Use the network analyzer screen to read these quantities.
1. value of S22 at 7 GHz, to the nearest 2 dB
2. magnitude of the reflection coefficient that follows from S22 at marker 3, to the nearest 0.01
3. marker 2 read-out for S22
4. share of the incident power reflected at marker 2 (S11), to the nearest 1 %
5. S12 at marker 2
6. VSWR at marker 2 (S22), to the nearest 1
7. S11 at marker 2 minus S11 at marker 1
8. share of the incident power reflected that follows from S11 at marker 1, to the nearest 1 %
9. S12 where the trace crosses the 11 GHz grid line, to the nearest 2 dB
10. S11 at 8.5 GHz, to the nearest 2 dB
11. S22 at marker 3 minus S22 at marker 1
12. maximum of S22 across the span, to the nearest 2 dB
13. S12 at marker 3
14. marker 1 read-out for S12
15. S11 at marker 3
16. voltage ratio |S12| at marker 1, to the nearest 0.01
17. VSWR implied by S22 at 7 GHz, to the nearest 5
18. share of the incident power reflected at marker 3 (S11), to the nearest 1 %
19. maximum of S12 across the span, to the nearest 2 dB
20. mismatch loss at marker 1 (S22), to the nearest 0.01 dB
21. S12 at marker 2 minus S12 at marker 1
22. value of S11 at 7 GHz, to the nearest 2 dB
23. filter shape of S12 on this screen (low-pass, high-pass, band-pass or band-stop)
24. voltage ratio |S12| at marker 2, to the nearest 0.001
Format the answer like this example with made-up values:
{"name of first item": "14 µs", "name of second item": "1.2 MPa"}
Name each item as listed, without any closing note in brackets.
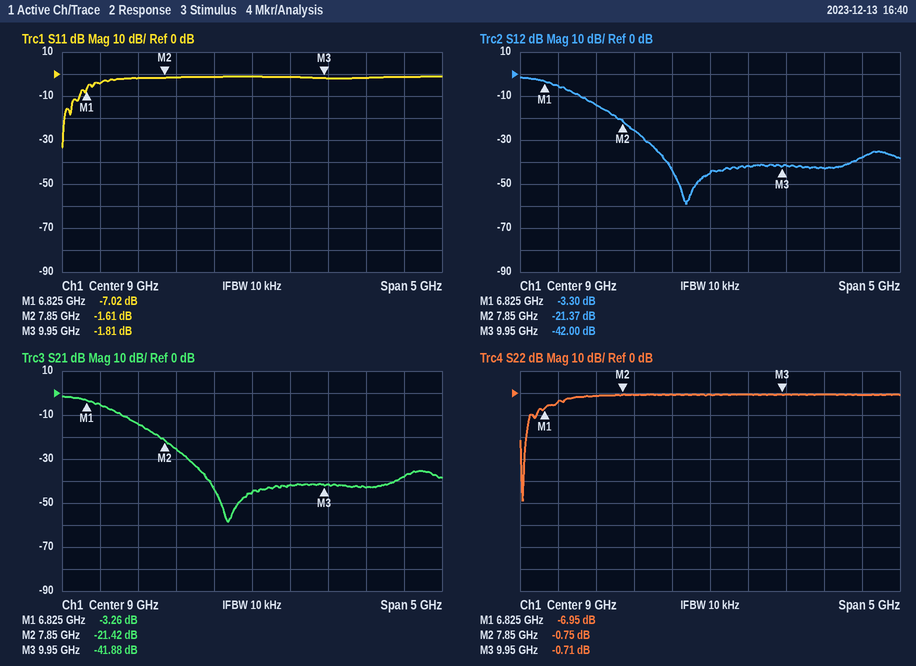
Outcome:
{"value of S22 at 7 GHz, to the nearest 2 dB": "-4 dB", "magnitude of the reflection coefficient that follows from S22 at marker 3, to the nearest 0.01": "0.92", "marker 2 read-out for S22": "-0.75 dB", "share of the incident power reflected at marker 2 (S11), to the nearest 1 %": "69 %", "S12 at marker 2": "-21.37 dB", "VSWR at marker 2 (S22), to the nearest 1": "23", "S11 at marker 2 minus S11 at marker 1": "5.41 dB", "share of the incident power reflected that follows from S11 at marker 1, to the nearest 1 %": "20 %", "S12 where the trace crosses the 11 GHz grid line, to the nearest 2 dB": "-38 dB", "S11 at 8.5 GHz, to the nearest 2 dB": "-2 dB", "S22 at marker 3 minus S22 at marker 1": "6.24 dB", "maximum of S22 across the span, to the nearest 2 dB": "0 dB", "S12 at marker 3": "-42.00 dB", "marker 1 read-out for S12": "-3.30 dB", "S11 at marker 3": "-1.81 dB", "voltage ratio |S12| at marker 1, to the nearest 0.01": "0.68", "VSWR implied by S22 at 7 GHz, to the nearest 5": "5", "share of the incident power reflected at marker 3 (S11), to the nearest 1 %": "66 %", "maximum of S12 across the span, to the nearest 2 dB": "-2 dB", "mismatch loss at marker 1 (S22), to the nearest 0.01 dB": "0.98 dB", "S12 at marker 2 minus S12 at marker 1": "-18.07 dB", "value of S11 at 7 GHz, to the nearest 2 dB": "-4 dB", "filter shape of S12 on this screen": "low-pass", "voltage ratio |S12| at marker 2, to the nearest 0.001": "0.085"}
